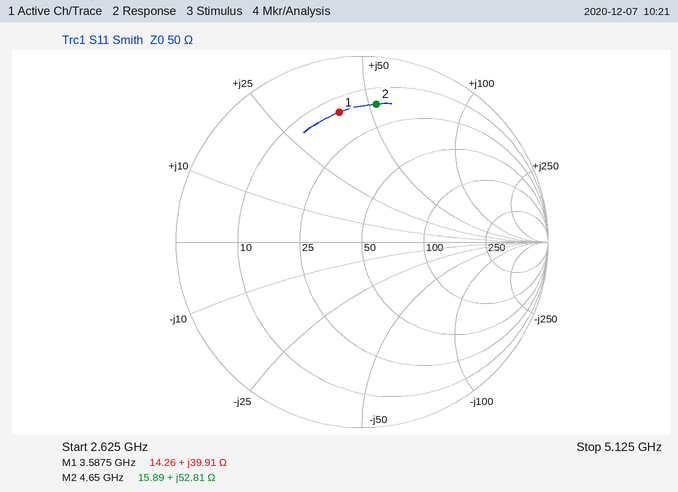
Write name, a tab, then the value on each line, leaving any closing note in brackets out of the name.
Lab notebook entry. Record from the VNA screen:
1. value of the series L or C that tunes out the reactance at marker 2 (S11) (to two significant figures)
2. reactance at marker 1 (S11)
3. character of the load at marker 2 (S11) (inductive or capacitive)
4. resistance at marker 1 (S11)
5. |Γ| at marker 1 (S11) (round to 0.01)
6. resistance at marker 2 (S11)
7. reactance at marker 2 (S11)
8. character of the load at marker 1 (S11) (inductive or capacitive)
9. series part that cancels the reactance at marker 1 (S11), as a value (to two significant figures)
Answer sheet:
value of the series L or C that tunes out the reactance at marker 2 (S11)	650 fF
reactance at marker 1	+39.91 Ω
character of the load at marker 2 (S11)	inductive
resistance at marker 1	14.26 Ω
|Γ| at marker 1 (S11)	0.71
resistance at marker 2	15.89 Ω
reactance at marker 2	+52.81 Ω
character of the load at marker 1 (S11)	inductive
series part that cancels the reactance at marker 1 (S11), as a value	1.1 pF
